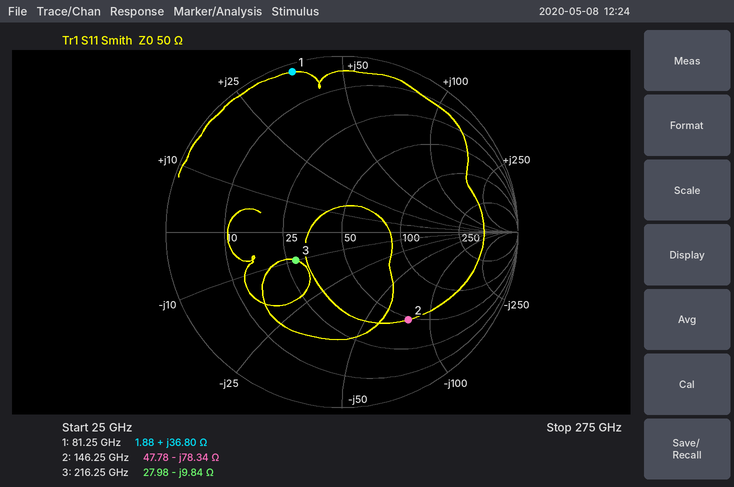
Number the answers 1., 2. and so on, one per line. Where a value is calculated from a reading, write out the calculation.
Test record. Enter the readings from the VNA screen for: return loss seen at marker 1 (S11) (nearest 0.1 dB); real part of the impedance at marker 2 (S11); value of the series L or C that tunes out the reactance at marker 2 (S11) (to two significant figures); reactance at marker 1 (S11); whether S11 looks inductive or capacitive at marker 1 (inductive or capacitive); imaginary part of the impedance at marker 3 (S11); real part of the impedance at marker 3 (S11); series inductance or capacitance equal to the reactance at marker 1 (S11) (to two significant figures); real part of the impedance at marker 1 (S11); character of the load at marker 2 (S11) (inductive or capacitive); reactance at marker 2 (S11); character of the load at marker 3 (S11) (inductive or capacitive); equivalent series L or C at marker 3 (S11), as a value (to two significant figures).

1. 0.4 dB
2. 47.78 Ω
3. L = 78.34 Ω/(2π × 146.25 GHz) ≈ 85 pH
4. +36.80 Ω
5. inductive
6. -9.84 Ω
7. 27.98 Ω
8. L = 36.8 Ω/(2π × 81.25 GHz) ≈ 72 pH
9. 1.88 Ω
10. capacitive
11. -78.34 Ω
12. capacitive
13. C = 1/(2π × 216.25 GHz × 9.84 Ω) ≈ 75 fF
